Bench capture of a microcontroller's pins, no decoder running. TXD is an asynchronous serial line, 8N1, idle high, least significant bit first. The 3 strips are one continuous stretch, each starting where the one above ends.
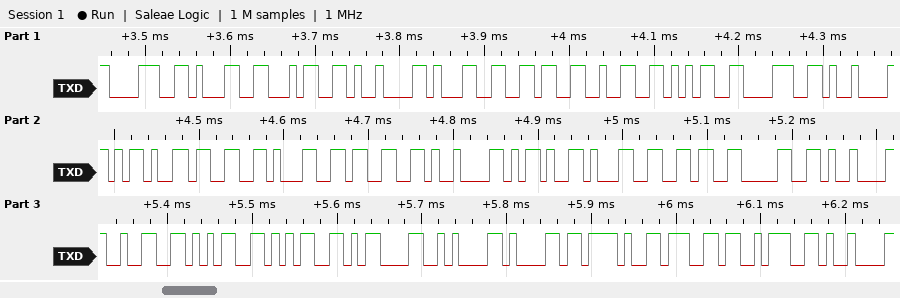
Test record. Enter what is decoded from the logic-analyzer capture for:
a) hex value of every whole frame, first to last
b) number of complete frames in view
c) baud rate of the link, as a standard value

38 31 34 09 31 36 32 35 38 09 2D 33 31 33 09 2D 31 36 30 09 32 35 35 0D 0A 61 2F 67 3A 09
30
115200 baud
